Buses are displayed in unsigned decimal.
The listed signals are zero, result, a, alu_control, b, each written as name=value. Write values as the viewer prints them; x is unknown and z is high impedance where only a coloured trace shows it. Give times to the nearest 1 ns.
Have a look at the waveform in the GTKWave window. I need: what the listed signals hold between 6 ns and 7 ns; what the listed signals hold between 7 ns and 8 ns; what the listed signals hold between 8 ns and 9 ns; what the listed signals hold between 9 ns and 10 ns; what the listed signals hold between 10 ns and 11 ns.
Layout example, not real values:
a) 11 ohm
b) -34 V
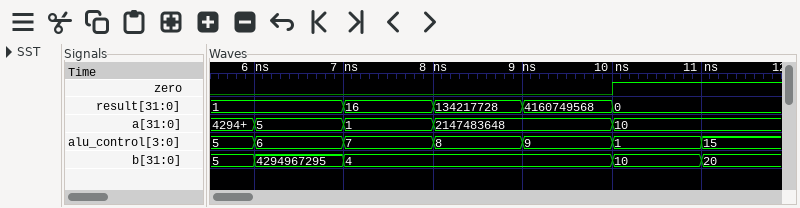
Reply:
a) zero=0, result=1, a=5, alu_control=6, b=4294967295
b) zero=0, result=16, a=1, alu_control=7, b=4
c) zero=0, result=134217728, a=2147483648, alu_control=8, b=4
d) zero=0, result=4160749568, a=2147483648, alu_control=9, b=4
e) zero=1, result=0, a=10, alu_control=1, b=10
